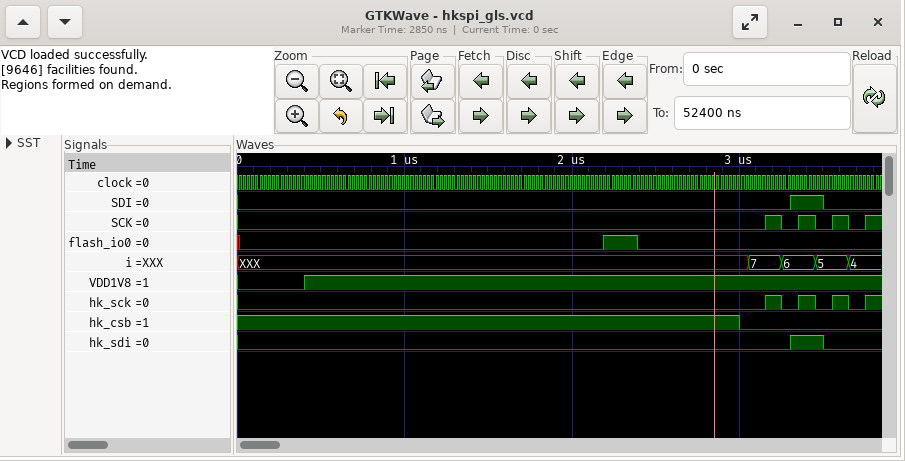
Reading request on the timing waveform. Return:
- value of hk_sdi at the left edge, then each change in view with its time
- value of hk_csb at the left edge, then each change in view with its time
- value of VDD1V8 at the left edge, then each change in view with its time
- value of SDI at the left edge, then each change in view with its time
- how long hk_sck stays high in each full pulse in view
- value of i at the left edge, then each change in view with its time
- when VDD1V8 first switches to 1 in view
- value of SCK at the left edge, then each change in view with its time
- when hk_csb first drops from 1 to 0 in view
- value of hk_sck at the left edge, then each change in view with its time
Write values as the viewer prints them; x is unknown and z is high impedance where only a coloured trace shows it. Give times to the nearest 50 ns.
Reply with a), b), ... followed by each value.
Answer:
a) 0, 1 at 3300 ns, 0 at 3500 ns
b) 1, 0 at 3000 ns
c) 0, 1 at 400 ns
d) 0, 1 at 3300 ns, 0 at 3500 ns
e) 100 ns, 100 ns, 100 ns
f) XXX, 7 at 3050 ns, 6 at 3250 ns, 5 at 3450 ns, 4 at 3650 ns
g) 400 ns
h) 0, 1 at 3150 ns, 0 at 3250 ns, 1 at 3350 ns, 0 at 3450 ns, 1 at 3550 ns, 0 at 3650 ns, 1 at 3750 ns
i) 3000 ns
j) 0, 1 at 3150 ns, 0 at 3250 ns, 1 at 3350 ns, 0 at 3450 ns, 1 at 3550 ns, 0 at 3650 ns, 1 at 3750 ns
